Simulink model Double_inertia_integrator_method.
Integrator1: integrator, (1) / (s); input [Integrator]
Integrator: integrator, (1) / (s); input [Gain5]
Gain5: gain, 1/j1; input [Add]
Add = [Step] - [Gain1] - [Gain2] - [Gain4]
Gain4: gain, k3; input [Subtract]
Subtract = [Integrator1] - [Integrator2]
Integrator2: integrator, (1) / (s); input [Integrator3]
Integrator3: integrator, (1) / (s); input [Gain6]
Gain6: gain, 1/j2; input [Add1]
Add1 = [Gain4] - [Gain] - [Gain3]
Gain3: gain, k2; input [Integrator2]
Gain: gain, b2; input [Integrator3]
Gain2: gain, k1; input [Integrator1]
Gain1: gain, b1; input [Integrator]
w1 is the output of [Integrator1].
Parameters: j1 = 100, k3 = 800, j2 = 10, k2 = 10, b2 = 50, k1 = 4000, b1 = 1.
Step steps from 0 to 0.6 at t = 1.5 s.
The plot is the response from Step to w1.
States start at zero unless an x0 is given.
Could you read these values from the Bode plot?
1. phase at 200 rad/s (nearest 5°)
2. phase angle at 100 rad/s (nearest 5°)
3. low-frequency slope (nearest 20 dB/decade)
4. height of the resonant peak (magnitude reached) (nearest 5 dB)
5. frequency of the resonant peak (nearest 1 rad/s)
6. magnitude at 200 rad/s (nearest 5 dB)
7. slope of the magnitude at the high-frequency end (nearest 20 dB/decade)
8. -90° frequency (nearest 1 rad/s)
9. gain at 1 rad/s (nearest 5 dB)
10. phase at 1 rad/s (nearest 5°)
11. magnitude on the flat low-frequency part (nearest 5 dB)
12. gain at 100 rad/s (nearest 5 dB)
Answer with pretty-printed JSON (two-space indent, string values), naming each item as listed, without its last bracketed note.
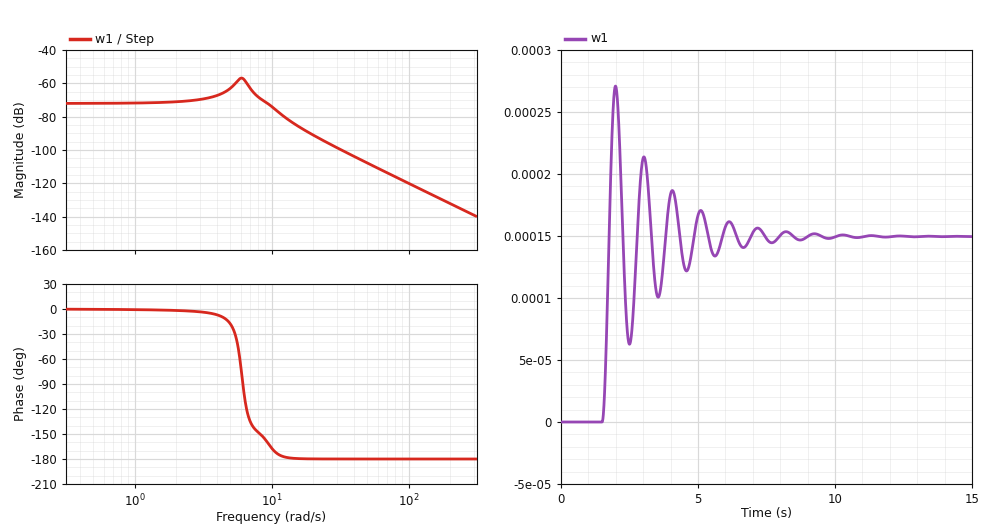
{
  "phase at 200 rad/s": "-180°",
  "phase angle at 100 rad/s": "-180°",
  "low-frequency slope": "0 dB/decade",
  "height of the resonant peak (magnitude reached)": "-55 dB",
  "frequency of the resonant peak": "6 rad/s",
  "magnitude at 200 rad/s": "-130 dB",
  "slope of the magnitude at the high-frequency end": "-40 dB/decade",
  "-90° frequency": "6 rad/s",
  "gain at 1 rad/s": "-70 dB",
  "phase at 1 rad/s": "0°",
  "magnitude on the flat low-frequency part": "-70 dB",
  "gain at 100 rad/s": "-120 dB"
}
